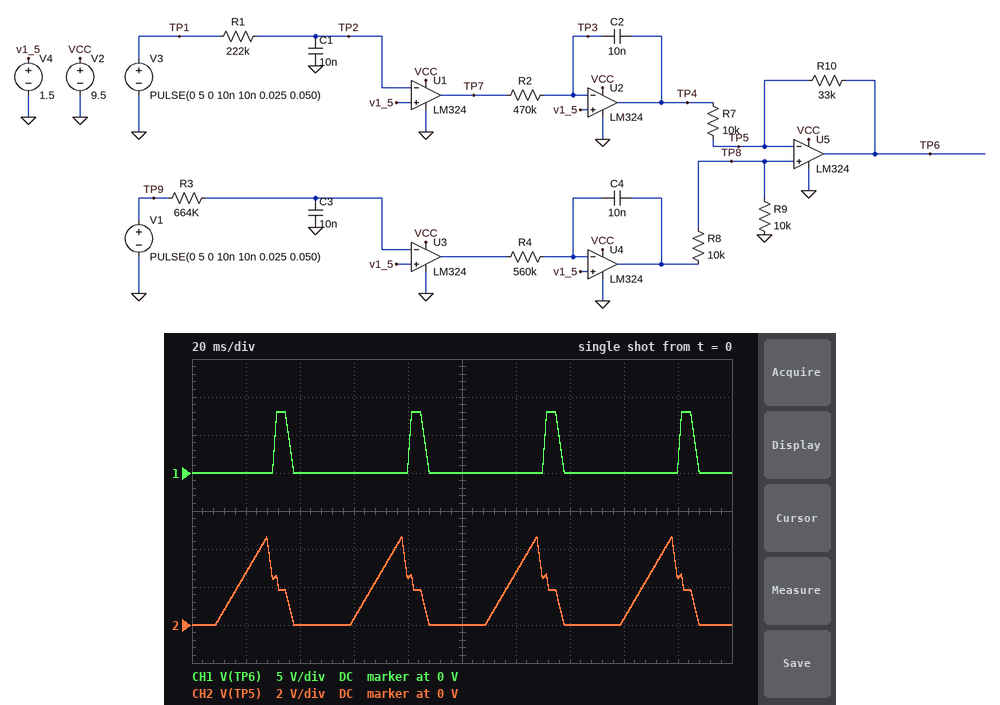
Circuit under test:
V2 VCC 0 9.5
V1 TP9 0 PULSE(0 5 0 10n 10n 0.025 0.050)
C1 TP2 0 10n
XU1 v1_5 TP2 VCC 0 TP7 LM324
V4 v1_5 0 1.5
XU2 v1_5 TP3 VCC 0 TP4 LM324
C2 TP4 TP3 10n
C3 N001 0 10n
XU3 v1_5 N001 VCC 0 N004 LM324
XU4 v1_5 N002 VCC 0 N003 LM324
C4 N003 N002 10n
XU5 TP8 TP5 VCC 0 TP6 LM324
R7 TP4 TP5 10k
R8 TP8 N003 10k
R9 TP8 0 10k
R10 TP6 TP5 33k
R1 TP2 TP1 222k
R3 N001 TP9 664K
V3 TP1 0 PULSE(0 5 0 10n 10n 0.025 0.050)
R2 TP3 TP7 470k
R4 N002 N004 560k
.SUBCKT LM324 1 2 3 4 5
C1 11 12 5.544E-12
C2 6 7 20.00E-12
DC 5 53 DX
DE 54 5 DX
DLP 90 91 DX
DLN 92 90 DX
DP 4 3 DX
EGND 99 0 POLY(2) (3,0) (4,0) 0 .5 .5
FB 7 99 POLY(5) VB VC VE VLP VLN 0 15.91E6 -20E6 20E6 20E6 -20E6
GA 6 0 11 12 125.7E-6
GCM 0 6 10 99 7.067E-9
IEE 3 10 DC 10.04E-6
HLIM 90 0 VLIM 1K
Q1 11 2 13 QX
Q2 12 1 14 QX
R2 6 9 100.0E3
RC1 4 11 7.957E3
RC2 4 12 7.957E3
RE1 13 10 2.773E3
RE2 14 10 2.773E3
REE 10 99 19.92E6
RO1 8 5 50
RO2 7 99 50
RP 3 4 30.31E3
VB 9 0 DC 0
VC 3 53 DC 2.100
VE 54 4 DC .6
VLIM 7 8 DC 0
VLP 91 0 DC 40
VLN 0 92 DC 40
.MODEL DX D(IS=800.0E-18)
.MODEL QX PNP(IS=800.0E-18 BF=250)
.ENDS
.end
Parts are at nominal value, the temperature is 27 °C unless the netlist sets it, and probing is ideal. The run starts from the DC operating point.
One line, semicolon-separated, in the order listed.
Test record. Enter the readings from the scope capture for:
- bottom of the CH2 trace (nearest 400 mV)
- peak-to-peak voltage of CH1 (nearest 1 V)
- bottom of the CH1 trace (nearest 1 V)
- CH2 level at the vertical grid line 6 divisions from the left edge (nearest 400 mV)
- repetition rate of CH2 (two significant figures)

0 V; 8 V; 0 V; 2.8 V; 20 Hz
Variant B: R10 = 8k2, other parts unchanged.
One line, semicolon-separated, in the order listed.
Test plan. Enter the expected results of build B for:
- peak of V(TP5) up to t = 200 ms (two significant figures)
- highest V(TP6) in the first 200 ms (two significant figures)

2.9 V; 5.2 V
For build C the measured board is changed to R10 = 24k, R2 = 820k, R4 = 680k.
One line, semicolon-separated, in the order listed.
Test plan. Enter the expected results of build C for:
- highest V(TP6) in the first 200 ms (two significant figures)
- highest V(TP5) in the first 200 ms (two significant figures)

7.4 V; 2.2 V
